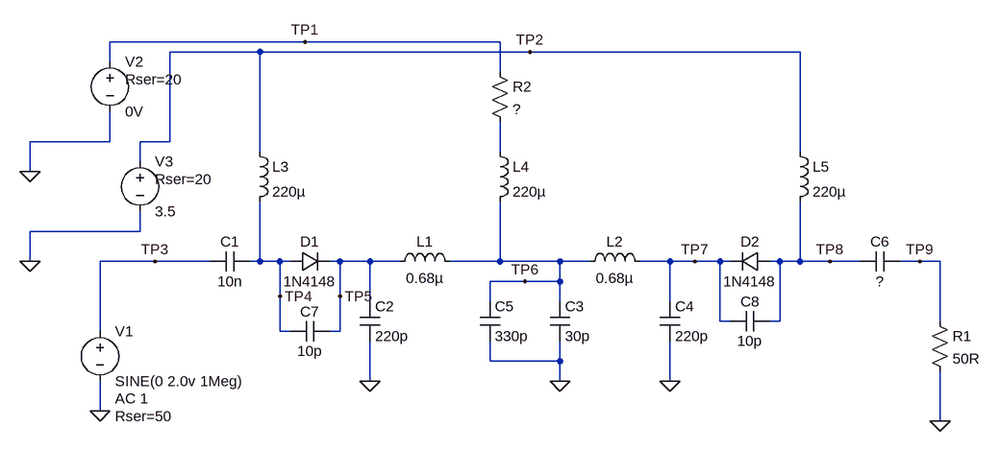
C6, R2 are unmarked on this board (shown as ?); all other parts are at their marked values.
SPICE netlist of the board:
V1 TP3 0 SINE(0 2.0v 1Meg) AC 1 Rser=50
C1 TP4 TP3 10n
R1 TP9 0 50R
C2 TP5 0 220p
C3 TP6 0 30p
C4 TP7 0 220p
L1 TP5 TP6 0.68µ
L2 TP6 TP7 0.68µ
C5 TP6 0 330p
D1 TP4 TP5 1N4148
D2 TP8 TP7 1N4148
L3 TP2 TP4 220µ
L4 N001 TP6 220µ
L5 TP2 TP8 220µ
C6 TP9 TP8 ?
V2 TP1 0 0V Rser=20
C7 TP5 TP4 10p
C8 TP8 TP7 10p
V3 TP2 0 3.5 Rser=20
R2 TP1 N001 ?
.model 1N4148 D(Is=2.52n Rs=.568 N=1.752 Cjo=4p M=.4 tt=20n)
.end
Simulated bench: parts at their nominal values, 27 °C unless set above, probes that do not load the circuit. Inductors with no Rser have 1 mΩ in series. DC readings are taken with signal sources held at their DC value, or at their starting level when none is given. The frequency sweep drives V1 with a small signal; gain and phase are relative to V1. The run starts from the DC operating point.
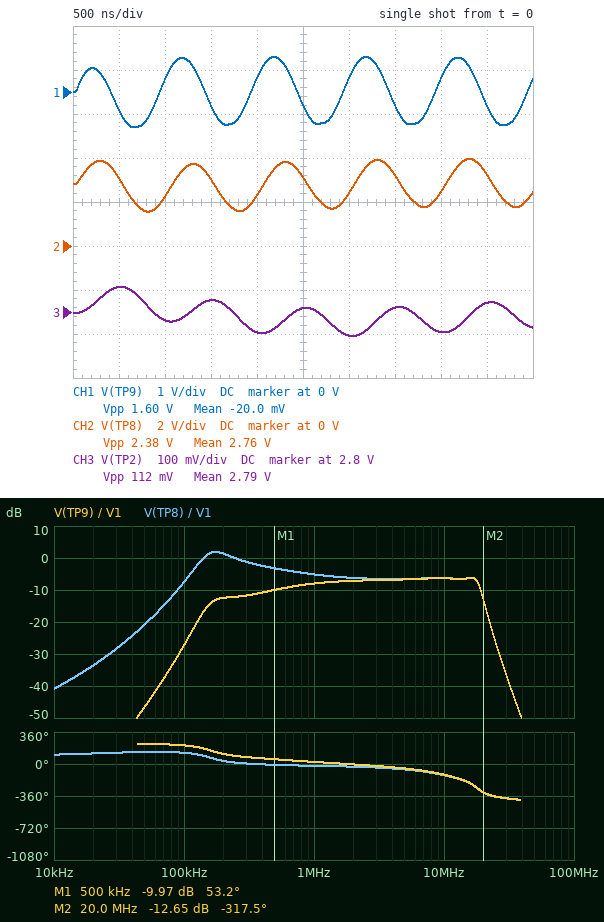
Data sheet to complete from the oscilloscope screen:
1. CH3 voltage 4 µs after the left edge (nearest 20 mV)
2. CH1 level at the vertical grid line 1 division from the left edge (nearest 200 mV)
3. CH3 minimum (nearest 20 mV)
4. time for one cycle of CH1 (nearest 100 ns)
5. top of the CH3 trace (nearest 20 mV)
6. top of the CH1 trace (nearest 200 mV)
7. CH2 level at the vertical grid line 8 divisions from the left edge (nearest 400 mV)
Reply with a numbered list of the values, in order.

1. 2.76 V
2. -400 mV
3. 2.74 V
4. 1.0 µs
5. 2.86 V
6. 800 mV
7. 2.4 V
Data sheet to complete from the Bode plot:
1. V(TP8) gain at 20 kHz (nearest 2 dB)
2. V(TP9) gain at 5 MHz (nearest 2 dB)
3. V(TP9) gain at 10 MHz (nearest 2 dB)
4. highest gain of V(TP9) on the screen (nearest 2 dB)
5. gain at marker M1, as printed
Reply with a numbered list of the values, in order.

1. -34 dB
2. -6 dB
3. -6 dB
4. -6 dB
5. -9.97 dB
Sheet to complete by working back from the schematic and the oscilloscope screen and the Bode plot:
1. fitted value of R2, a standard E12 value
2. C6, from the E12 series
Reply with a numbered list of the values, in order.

1. 39 Ω
2. 3.3 nF
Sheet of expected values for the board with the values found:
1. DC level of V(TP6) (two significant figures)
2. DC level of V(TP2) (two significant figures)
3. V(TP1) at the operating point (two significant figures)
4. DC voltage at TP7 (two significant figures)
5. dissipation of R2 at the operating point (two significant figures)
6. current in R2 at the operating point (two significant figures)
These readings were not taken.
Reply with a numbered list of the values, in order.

1. 2.1 V
2. 2.8 V
3. 700 mV
4. 2.1 V
5. 48 mW
6. 35 mA
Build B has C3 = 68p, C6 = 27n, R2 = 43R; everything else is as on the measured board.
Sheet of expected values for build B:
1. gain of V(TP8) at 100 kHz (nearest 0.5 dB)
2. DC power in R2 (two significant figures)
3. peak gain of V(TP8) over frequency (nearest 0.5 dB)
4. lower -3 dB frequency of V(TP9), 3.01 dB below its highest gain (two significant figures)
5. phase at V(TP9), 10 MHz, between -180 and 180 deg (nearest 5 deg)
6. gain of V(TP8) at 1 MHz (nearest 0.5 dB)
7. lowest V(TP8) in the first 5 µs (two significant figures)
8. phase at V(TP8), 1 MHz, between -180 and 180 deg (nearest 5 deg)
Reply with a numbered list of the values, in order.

1. -9.5 dB
2. 48 mW
3. -6.0 dB
4. 160 kHz
5. -125 deg
6. -6.5 dB
7. 2.0 V
8. -5 deg
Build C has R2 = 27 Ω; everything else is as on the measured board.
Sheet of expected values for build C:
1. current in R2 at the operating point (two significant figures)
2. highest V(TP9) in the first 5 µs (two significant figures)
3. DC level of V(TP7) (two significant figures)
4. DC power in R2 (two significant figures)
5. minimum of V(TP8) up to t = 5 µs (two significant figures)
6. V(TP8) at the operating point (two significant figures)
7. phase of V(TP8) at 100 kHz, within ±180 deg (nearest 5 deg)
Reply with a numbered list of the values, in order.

1. 41 mA
2. 810 mV
3. 1.9 V
4. 46 mW
5. 1.4 V
6. 2.7 V
7. 130 deg
